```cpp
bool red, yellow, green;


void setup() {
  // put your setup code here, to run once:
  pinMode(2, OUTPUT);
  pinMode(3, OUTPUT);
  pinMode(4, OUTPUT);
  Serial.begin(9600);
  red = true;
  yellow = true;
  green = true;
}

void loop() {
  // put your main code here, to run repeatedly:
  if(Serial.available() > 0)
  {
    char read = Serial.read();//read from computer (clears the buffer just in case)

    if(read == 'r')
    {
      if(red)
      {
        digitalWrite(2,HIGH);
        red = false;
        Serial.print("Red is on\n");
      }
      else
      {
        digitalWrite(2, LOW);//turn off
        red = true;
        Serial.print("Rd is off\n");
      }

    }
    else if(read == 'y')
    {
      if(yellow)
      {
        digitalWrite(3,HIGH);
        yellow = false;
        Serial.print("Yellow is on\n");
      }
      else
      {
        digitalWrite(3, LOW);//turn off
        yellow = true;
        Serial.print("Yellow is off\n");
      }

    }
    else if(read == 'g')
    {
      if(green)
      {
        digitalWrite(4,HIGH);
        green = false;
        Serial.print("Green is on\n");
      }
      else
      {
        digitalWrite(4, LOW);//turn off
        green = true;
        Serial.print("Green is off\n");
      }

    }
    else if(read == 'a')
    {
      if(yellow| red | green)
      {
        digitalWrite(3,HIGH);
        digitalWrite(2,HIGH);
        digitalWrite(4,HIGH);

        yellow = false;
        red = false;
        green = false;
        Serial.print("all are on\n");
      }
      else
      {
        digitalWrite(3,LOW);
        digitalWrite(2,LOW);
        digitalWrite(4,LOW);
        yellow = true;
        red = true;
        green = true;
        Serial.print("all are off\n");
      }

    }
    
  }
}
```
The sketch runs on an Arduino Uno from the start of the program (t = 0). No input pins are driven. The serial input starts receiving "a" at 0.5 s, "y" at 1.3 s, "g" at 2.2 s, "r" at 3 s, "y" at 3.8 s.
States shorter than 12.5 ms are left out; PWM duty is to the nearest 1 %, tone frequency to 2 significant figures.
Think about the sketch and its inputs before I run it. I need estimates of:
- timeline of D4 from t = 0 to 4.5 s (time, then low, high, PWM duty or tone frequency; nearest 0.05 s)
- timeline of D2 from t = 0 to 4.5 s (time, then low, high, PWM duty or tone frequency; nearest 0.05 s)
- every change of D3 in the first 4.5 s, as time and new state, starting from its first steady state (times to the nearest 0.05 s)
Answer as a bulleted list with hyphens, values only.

- 0 s low; 0.5 s high; 2.2 s low
- 0 s low; 0.5 s high; 3 s low
- 0 s low; 0.5 s high; 1.3 s low; 3.8 s high
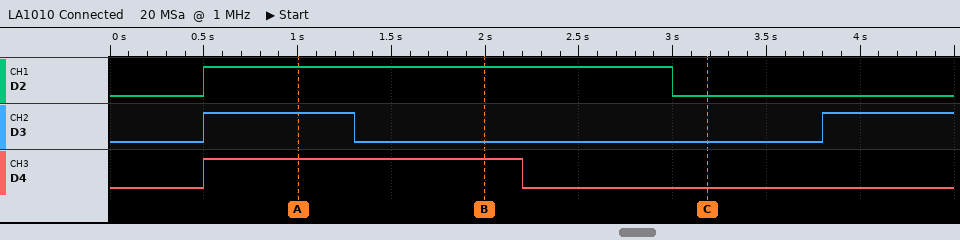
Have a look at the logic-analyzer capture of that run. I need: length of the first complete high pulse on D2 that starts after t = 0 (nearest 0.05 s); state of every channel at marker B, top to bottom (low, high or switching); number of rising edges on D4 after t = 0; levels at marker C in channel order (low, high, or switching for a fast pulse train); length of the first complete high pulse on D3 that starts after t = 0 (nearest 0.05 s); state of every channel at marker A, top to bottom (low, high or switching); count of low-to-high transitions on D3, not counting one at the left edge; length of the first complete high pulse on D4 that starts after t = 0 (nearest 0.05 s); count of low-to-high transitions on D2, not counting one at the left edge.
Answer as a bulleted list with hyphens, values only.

- 2.50 s
- D2 high, D3 low, D4 high
- 1
- D2 low, D3 low, D4 low
- 0.80 s
- D2 high, D3 high, D4 high
- 2
- 1.70 s
- 1
